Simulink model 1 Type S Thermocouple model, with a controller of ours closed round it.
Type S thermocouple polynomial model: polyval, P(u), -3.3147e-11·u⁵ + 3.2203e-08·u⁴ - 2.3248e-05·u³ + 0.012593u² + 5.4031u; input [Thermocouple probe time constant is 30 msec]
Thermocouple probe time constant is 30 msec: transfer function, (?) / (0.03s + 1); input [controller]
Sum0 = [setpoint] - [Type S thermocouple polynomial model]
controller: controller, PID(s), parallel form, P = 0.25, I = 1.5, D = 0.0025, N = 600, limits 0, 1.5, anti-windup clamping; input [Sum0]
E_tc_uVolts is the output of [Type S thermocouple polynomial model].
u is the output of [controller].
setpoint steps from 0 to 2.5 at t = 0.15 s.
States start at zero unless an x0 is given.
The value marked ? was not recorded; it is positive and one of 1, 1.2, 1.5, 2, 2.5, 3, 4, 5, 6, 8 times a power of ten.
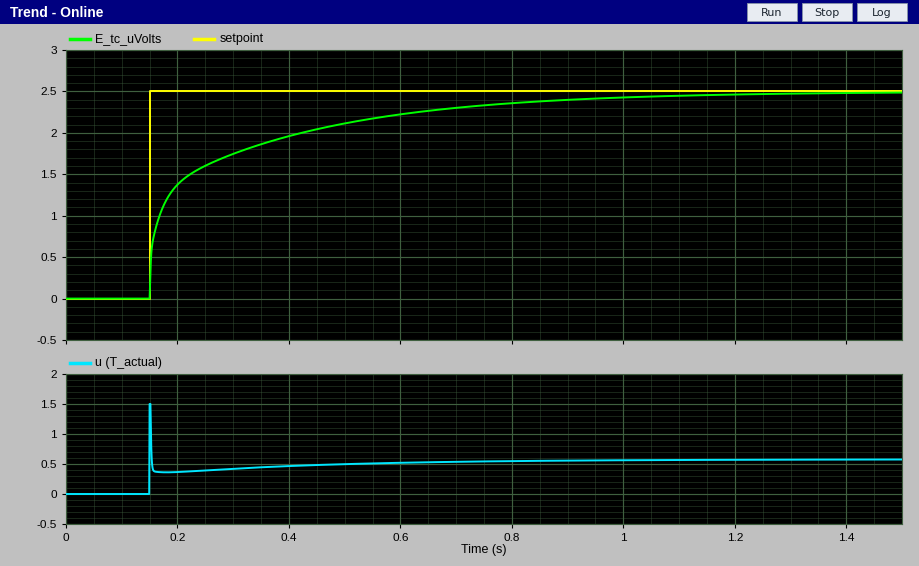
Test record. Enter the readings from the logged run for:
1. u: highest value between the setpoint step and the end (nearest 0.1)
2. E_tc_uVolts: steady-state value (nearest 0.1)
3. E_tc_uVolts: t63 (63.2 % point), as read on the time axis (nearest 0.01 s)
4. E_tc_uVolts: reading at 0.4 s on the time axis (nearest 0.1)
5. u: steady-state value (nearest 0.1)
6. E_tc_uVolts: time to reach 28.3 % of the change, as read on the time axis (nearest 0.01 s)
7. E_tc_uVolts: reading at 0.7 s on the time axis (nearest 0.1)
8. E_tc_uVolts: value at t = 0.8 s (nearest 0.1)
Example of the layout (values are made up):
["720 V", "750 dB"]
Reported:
["1.5", "2.5", "0.24 s", "2.0", "0.6", "0.16 s", "2.3", "2.4"]
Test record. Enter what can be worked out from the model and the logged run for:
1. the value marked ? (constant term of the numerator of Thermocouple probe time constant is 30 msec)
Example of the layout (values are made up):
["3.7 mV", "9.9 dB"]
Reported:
["0.8"]
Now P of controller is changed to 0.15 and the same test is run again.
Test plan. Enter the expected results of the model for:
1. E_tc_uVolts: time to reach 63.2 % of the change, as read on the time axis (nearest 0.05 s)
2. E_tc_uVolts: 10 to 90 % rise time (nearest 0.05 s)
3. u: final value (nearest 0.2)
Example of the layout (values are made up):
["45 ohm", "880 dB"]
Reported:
["0.30 s", "0.45 s", "0.6"]
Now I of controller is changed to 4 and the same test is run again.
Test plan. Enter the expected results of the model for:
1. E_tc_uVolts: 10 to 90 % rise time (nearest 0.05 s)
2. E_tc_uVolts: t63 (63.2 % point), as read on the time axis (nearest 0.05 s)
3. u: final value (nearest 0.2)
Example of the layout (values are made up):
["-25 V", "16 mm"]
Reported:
["0.15 s", "0.20 s", "0.6"]
